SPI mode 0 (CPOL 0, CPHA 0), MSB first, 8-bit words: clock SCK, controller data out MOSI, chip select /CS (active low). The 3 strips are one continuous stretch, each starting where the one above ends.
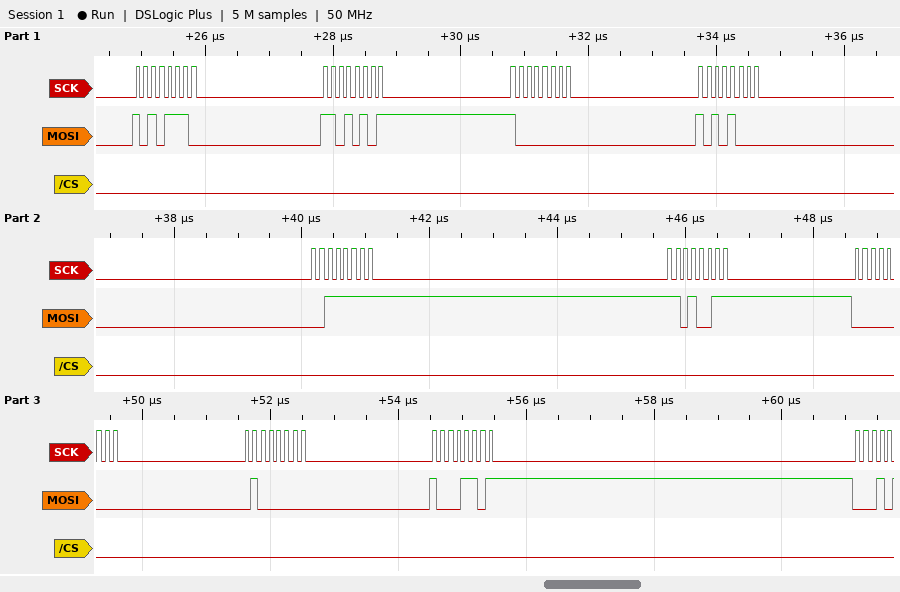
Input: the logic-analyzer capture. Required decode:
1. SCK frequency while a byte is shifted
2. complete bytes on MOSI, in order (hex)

8 MHz
AE D5 80 A8 3F D3 00 40 8D
